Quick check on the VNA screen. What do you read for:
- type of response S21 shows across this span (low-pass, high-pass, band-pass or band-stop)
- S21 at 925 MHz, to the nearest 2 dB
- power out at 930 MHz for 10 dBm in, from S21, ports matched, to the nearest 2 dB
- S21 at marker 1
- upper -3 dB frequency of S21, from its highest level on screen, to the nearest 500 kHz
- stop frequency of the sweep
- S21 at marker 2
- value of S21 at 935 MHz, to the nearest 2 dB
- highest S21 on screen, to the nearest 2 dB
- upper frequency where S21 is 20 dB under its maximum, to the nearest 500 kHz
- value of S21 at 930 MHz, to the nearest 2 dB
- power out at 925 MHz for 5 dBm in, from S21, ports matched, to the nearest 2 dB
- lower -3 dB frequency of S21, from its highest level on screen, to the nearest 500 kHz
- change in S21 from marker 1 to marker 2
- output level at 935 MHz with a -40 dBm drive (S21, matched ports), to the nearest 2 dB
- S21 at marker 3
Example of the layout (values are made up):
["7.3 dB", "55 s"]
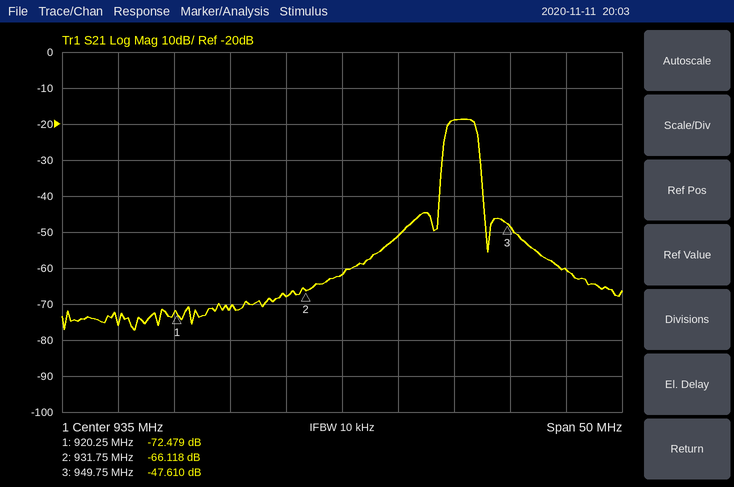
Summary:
["band-pass", "-72 dB", "-58 dBm", "-72.479 dB", "947.0 MHz", "960 MHz", "-66.118 dB", "-62 dB", "-18 dB", "947.5 MHz", "-68 dB", "-66 dBm", "944.5 MHz", "6.361 dB", "-102 dBm", "-47.610 dB"]
